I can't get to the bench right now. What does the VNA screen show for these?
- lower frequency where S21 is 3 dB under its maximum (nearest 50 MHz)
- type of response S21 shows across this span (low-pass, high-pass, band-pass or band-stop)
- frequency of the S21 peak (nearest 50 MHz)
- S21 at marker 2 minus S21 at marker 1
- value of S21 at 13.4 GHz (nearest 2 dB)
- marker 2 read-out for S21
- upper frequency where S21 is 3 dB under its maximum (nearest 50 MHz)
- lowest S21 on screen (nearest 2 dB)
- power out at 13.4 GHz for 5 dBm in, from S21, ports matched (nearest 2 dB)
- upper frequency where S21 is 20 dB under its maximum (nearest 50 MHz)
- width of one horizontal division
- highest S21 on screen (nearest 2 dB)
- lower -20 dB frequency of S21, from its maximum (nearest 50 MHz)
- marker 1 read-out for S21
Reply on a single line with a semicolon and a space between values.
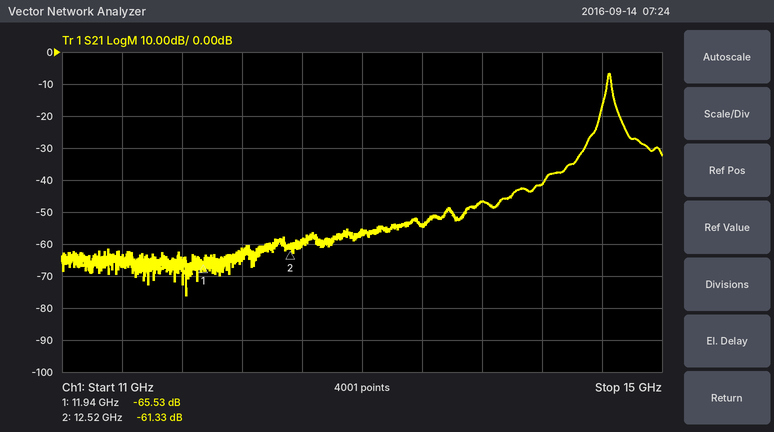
14.65 GHz; band-pass; 14.65 GHz; 4.20 dB; -54 dB; -61.33 dB; 14.65 GHz; -76 dB; -50 dBm; 14.80 GHz; 400 MHz; -6 dB; 14.50 GHz; -65.53 dB
